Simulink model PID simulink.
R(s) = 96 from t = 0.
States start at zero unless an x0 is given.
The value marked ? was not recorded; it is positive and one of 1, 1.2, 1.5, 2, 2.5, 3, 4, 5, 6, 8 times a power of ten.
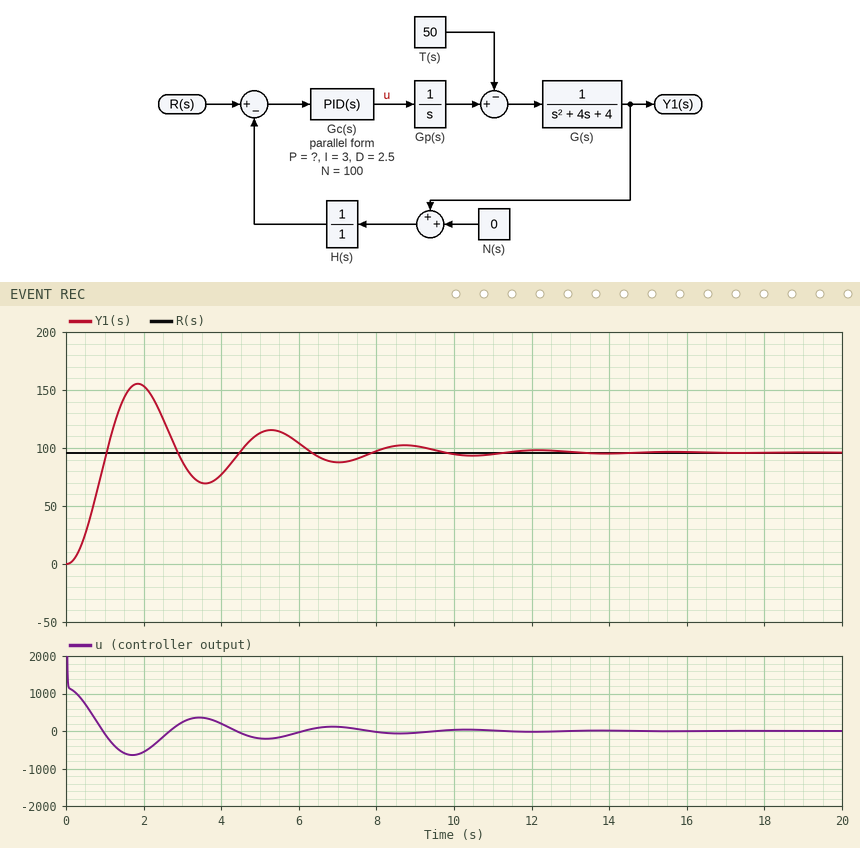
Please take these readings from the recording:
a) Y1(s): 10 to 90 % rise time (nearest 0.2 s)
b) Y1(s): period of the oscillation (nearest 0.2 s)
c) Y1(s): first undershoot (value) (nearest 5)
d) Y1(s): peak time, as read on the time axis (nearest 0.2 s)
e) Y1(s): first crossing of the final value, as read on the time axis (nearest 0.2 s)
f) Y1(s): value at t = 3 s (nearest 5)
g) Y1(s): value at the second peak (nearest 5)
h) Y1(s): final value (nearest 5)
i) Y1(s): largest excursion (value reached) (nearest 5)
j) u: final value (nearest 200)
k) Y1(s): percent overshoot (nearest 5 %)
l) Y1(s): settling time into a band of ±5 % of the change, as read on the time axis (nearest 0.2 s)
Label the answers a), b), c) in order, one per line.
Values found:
a) 0.6 s
b) 3.4 s
c) 70
d) 1.8 s
e) 1.0 s
f) 90
g) 115
h) 95
i) 155
j) 0
k) 60 %
l) 9.2 s
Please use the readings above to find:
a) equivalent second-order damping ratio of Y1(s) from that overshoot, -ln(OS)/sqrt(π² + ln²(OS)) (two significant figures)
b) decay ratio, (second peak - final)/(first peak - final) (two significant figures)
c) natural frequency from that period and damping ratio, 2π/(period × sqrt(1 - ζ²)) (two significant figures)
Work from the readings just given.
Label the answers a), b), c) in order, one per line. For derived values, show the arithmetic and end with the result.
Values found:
a) ln(0.6) = -0.511; 0.511 / sqrt(9.870 + 0.261) = 0.16
b) (115 - 95) / (155 - 95) = 0.33
c) 2π / (3.4 × sqrt(1 - 0.16²)) = 1.9 rad/s
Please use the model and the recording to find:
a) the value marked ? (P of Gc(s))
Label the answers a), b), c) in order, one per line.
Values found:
a) 12
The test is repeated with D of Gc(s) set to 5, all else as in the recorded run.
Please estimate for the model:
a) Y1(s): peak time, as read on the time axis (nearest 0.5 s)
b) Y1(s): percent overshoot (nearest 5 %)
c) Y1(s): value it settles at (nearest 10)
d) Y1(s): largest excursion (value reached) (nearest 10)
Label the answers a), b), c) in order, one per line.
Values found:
a) 1.5 s
b) 40 %
c) 100
d) 130
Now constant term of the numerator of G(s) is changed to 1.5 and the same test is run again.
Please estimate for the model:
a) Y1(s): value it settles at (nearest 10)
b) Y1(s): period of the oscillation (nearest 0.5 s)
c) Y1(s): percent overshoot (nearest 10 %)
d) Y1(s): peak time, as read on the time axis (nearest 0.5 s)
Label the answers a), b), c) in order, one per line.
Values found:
a) 100
b) 3.0 s
c) 70 %
d) 1.5 s
